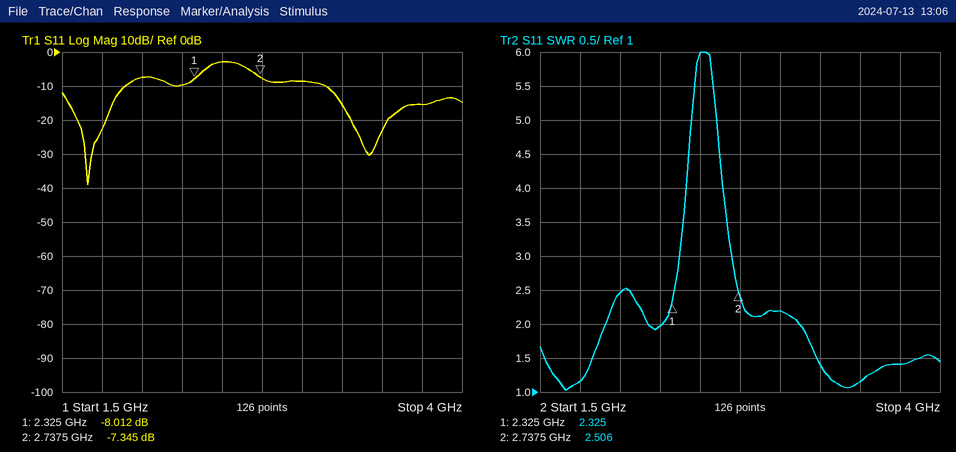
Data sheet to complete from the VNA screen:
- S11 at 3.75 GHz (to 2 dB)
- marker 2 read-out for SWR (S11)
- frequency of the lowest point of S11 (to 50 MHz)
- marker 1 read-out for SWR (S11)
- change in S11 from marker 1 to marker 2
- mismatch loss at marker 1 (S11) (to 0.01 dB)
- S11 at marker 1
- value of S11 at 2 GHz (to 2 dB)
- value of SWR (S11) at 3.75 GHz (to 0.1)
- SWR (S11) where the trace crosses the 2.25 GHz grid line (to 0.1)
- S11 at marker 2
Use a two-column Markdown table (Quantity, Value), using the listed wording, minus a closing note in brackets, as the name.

| Quantity | Value |
|---|---|
| S11 at 3.75 GHz | -16 dB |
| marker 2 read-out for SWR | 2.506 |
| frequency of the lowest point of S11 | 1.65 GHz |
| marker 1 read-out for SWR | 2.325 |
| change in S11 from marker 1 to marker 2 | 0.667 dB |
| mismatch loss at marker 1 (S11) | 0.75 dB |
| S11 at marker 1 | -8.012 dB |
| value of S11 at 2 GHz | -8 dB |
| value of SWR (S11) at 3.75 GHz | 1.4 |
| SWR (S11) where the trace crosses the 2.25 GHz grid line | 2.0 |
| S11 at marker 2 | -7.345 dB |
